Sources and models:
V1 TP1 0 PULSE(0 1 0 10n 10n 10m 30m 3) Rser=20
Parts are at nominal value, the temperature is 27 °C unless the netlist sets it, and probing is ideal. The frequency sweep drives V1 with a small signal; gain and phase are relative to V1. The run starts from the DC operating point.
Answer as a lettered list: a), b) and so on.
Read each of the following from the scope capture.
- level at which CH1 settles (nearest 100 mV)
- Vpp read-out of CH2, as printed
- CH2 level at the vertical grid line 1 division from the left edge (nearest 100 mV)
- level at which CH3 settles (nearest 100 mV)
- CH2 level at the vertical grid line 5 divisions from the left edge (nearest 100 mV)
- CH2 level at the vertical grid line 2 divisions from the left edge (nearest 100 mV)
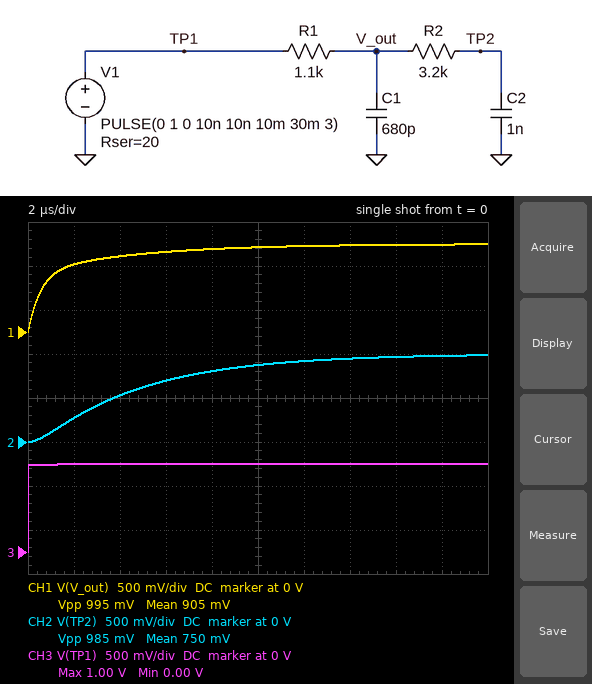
a) 1.0 V
b) 985 mV
c) 300 mV
d) 1.0 V
e) 900 mV
f) 500 mV
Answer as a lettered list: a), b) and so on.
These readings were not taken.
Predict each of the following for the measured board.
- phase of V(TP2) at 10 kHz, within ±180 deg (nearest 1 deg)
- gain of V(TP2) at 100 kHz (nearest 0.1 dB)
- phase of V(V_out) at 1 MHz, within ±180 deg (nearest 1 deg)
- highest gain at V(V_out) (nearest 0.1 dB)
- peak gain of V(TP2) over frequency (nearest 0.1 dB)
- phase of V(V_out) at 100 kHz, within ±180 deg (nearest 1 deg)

a) -18 deg
b) -10.1 dB
c) -74 deg
d) 0 dB
e) 0 dB
f) -26 deg
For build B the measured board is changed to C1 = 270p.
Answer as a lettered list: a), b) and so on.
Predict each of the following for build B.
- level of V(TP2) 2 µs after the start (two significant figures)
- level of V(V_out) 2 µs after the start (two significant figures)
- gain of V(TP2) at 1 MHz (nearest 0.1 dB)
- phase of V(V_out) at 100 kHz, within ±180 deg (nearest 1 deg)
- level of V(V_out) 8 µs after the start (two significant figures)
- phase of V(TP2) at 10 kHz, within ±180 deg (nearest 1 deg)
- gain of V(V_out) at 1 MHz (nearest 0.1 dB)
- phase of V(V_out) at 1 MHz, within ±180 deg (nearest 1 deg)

a) 330 mV
b) 820 mV
c) -33.5 dB
d) -14 deg
e) 950 mV
f) -16 deg
g) -7.4 dB
h) -55 deg
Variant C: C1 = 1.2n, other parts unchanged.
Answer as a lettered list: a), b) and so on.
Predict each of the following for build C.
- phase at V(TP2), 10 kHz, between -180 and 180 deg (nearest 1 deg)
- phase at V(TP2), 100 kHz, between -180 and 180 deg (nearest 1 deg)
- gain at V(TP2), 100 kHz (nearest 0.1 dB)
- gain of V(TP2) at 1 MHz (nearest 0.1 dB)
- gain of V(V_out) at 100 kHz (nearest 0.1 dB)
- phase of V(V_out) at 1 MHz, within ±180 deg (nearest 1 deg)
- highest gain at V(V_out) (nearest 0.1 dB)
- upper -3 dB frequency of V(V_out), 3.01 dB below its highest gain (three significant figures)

a) -20 deg
b) -101 deg
c) -11.2 dB
d) -44.7 dB
e) -4.2 dB
f) -81 deg
g) 0 dB
h) 64.7 kHz
